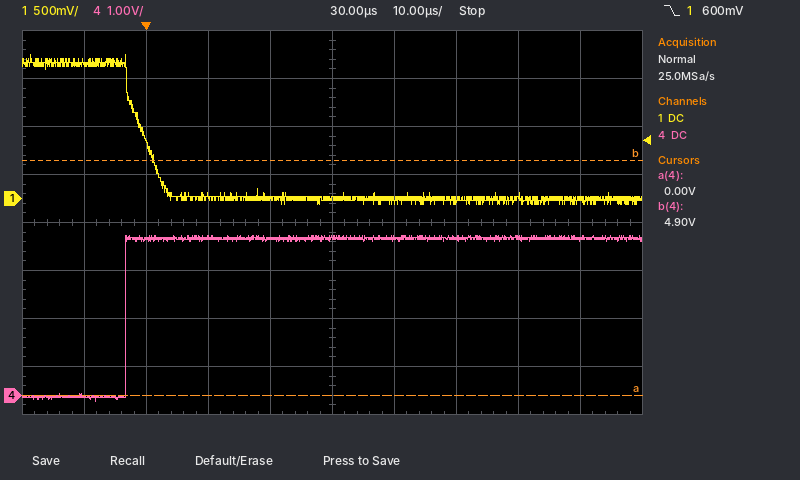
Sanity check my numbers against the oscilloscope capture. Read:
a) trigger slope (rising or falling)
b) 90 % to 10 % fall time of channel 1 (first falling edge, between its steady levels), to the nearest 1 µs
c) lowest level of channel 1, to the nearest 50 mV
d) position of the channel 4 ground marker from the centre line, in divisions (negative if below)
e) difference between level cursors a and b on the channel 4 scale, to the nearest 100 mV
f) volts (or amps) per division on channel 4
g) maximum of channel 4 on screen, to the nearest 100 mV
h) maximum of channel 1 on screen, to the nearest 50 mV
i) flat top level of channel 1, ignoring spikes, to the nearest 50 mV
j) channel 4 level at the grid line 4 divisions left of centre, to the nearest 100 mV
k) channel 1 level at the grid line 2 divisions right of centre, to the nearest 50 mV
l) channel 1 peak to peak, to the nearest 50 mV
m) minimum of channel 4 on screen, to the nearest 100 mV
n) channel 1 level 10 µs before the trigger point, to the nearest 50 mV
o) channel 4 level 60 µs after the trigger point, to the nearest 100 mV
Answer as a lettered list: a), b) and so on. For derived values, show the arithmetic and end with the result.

a) falling
b) 6 µs
c) -50 mV
d) -3.6 div
e) 4.9 V
f) 1 V
g) 3.3 V
h) 1.50 V
i) 1.40 V
j) 0.0 V
k) 0 mV
l) 1.50 V − (-50 mV) = 1.55 V
m) -100 mV
n) 1.40 V
o) 3.3 V
